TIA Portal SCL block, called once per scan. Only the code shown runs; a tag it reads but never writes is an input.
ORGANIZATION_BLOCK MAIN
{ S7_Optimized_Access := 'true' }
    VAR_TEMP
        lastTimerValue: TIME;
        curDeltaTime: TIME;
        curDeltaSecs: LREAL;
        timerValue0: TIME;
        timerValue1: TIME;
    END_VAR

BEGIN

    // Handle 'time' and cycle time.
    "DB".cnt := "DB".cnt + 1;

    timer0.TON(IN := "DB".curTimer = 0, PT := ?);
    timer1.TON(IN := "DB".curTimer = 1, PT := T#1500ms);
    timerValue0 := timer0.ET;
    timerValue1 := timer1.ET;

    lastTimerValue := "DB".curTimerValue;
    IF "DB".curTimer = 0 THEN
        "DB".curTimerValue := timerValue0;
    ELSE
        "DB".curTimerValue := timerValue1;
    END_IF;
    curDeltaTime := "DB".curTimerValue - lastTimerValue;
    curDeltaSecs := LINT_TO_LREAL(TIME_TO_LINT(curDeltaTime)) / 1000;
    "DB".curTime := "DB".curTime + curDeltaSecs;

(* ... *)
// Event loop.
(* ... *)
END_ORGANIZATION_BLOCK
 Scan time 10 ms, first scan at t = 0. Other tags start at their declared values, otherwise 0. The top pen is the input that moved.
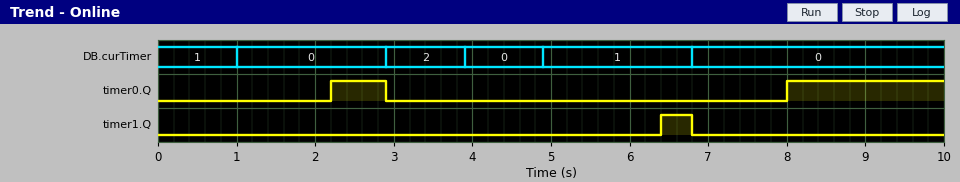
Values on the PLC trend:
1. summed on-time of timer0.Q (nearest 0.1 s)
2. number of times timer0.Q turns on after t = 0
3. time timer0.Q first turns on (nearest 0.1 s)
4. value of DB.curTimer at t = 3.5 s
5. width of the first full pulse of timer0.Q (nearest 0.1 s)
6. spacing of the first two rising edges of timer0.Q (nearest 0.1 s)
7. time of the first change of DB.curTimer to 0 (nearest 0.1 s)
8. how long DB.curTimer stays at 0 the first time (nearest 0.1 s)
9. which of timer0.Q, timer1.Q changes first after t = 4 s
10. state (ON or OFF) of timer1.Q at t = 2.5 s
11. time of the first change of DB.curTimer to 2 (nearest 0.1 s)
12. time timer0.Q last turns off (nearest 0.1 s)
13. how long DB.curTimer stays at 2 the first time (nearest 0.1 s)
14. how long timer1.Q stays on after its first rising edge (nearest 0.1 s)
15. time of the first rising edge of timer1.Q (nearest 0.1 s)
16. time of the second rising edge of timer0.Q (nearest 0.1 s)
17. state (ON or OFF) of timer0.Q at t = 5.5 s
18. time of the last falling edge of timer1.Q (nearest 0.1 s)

2.7 s
2
2.2 s
2
0.7 s
5.8 s
1.0 s
1.9 s
timer1.Q
OFF
2.9 s
2.9 s
1.0 s
0.4 s
6.4 s
8.0 s
OFF
6.8 s
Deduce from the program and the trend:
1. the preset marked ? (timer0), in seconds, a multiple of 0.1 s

1.2 s
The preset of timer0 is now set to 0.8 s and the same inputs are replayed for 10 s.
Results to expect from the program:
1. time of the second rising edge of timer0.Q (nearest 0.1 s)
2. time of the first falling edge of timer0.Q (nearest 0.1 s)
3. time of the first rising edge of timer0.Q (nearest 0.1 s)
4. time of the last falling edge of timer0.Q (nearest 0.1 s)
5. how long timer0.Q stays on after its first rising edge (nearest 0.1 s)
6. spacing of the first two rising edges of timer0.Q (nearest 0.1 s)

4.7 s
2.9 s
1.8 s
4.9 s
1.1 s
2.9 s
